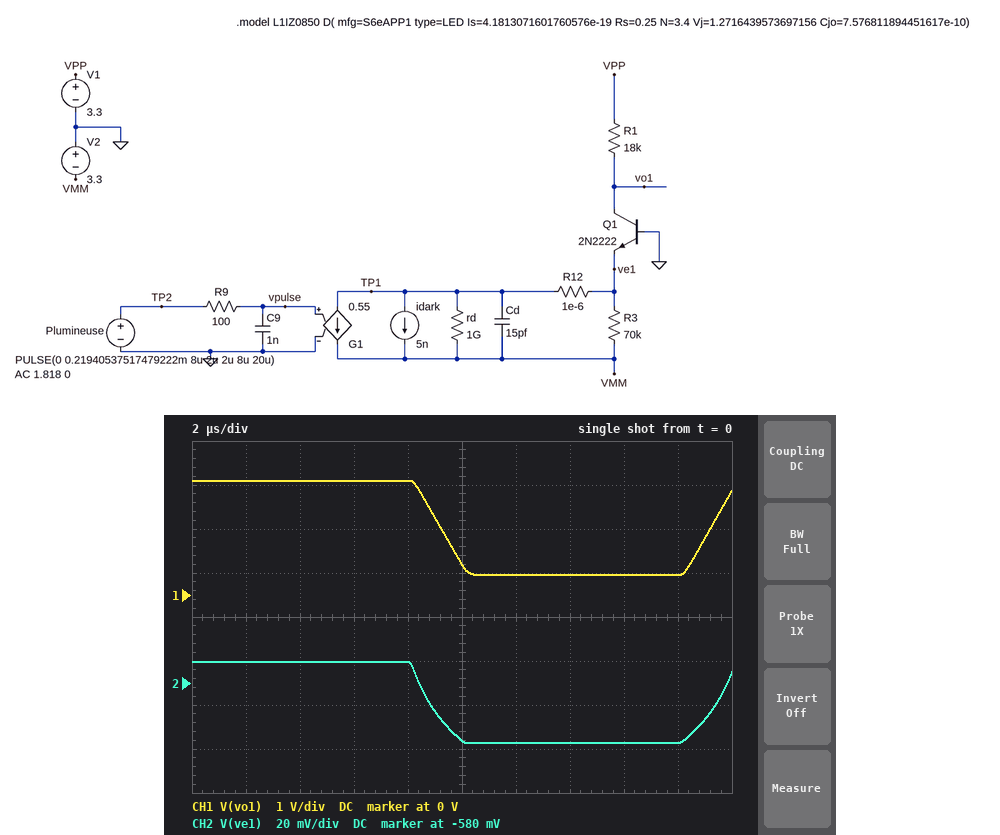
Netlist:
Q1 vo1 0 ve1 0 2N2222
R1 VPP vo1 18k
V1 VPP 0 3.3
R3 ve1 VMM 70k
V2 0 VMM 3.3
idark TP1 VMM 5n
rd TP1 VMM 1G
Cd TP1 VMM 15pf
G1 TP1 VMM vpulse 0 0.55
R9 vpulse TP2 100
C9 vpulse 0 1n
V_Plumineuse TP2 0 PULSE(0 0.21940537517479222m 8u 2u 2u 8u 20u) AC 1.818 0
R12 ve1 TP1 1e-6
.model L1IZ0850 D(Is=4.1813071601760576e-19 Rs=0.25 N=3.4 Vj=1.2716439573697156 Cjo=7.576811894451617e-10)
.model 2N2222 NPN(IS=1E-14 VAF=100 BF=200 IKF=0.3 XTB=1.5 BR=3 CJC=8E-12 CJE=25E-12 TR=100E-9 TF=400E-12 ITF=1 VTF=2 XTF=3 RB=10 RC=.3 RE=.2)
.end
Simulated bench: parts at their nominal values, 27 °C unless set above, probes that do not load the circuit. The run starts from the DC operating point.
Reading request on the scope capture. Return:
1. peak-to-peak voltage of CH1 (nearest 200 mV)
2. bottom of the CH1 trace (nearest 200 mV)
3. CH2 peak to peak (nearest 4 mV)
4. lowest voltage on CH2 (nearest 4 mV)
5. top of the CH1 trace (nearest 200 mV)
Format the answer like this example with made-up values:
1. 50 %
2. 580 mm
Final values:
1. 2.2 V
2. 400 mV
3. 36 mV
4. -608 mV
5. 2.6 V
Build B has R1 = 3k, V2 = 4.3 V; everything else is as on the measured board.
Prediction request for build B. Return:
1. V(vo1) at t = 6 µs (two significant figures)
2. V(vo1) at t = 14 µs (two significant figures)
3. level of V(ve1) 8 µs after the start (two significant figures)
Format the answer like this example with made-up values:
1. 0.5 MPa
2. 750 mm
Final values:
1. 3.1 V
2. 2.8 V
3. -580 mV
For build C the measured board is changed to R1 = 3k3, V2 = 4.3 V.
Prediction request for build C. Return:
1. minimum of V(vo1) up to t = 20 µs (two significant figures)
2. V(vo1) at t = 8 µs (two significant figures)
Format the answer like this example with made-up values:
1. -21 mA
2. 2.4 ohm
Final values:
1. 2.7 V
2. 3.1 V
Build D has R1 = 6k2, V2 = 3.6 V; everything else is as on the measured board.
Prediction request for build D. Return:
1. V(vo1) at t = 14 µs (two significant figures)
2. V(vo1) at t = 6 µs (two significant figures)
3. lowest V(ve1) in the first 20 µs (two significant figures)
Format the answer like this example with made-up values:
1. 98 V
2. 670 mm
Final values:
1. 2.3 V
2. 3.0 V
3. -610 mV
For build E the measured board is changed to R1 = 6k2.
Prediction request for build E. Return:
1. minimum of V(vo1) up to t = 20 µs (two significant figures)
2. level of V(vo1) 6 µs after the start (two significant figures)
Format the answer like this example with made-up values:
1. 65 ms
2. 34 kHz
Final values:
1. 2.3 V
2. 3.1 V
